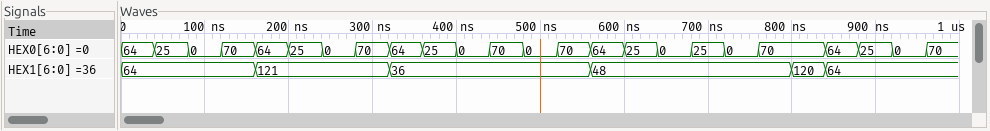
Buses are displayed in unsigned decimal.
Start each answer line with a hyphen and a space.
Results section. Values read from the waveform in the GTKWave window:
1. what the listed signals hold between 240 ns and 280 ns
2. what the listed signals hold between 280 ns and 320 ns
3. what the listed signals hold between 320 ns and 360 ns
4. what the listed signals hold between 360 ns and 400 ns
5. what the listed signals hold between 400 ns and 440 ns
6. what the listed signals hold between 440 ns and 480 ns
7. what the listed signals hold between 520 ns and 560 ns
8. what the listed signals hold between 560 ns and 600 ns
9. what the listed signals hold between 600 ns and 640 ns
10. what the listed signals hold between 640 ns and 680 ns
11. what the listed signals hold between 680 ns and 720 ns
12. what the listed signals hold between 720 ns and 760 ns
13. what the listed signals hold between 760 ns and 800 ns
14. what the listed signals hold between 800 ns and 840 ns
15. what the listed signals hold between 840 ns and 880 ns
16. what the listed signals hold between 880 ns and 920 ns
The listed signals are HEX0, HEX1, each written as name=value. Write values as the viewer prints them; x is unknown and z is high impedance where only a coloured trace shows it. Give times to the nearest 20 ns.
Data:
- HEX0=0, HEX1=121
- HEX0=70, HEX1=121
- HEX0=64, HEX1=36
- HEX0=25, HEX1=36
- HEX0=0, HEX1=36
- HEX0=70, HEX1=36
- HEX0=70, HEX1=36
- HEX0=64, HEX1=48
- HEX0=25, HEX1=48
- HEX0=0, HEX1=48
- HEX0=25, HEX1=48
- HEX0=0, HEX1=48
- HEX0=70, HEX1=48
- HEX0=70, HEX1=120
- HEX0=64, HEX1=64
- HEX0=25, HEX1=64
